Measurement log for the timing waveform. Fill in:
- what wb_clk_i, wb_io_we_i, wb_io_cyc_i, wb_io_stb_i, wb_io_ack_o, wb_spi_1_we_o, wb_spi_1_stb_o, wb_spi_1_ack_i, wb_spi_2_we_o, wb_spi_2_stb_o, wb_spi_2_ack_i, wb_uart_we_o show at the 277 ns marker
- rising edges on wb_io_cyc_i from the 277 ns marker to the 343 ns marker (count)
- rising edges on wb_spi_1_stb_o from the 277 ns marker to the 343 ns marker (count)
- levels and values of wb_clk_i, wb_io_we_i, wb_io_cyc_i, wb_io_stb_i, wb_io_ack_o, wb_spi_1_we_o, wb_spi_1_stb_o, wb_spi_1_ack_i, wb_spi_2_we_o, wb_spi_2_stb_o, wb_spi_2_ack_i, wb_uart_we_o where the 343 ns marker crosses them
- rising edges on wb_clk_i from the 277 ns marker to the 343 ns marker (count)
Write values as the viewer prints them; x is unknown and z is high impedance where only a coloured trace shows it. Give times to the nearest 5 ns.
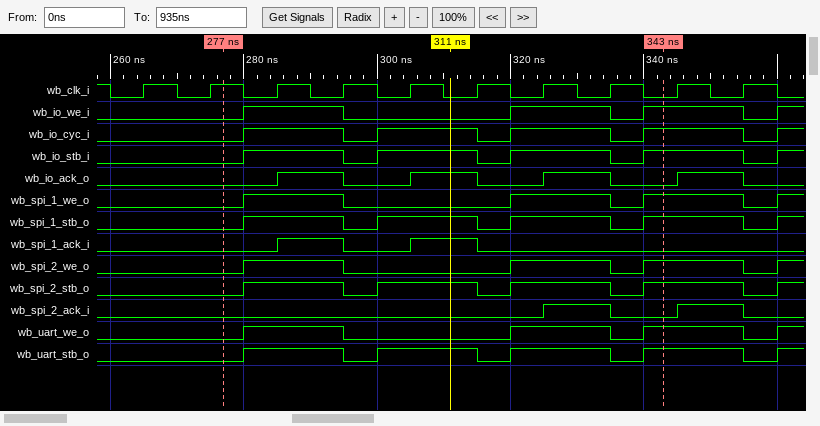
wb_clk_i=1, wb_io_we_i=0, wb_io_cyc_i=0, wb_io_stb_i=0, wb_io_ack_o=0, wb_spi_1_we_o=0, wb_spi_1_stb_o=0, wb_spi_1_ack_i=0, wb_spi_2_we_o=0, wb_spi_2_stb_o=0, wb_spi_2_ack_i=0, wb_uart_we_o=0
4
4
wb_clk_i=0, wb_io_we_i=1, wb_io_cyc_i=1, wb_io_stb_i=1, wb_io_ack_o=0, wb_spi_1_we_o=1, wb_spi_1_stb_o=1, wb_spi_1_ack_i=0, wb_spi_2_we_o=1, wb_spi_2_stb_o=1, wb_spi_2_ack_i=0, wb_uart_we_o=1
6
